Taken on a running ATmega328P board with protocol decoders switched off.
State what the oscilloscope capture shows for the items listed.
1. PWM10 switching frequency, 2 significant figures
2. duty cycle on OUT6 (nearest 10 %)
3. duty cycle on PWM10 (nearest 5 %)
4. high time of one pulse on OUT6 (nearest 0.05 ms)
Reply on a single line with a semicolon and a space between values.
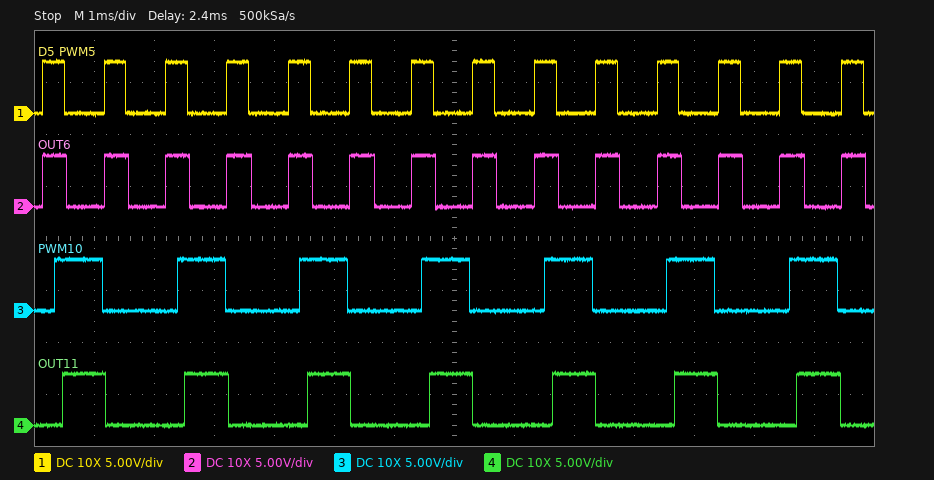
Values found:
490 Hz; 40 %; 40 %; 0.40 ms
